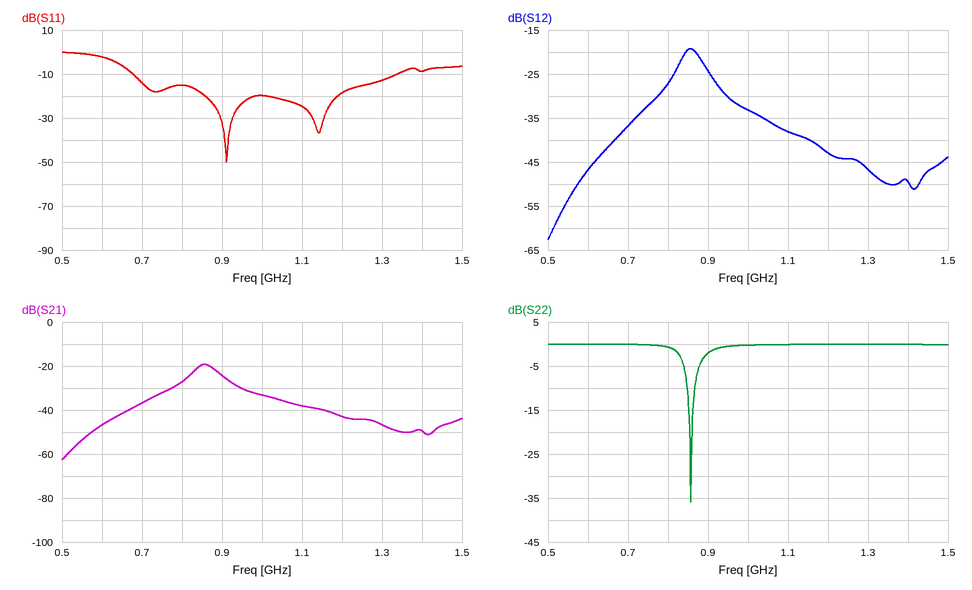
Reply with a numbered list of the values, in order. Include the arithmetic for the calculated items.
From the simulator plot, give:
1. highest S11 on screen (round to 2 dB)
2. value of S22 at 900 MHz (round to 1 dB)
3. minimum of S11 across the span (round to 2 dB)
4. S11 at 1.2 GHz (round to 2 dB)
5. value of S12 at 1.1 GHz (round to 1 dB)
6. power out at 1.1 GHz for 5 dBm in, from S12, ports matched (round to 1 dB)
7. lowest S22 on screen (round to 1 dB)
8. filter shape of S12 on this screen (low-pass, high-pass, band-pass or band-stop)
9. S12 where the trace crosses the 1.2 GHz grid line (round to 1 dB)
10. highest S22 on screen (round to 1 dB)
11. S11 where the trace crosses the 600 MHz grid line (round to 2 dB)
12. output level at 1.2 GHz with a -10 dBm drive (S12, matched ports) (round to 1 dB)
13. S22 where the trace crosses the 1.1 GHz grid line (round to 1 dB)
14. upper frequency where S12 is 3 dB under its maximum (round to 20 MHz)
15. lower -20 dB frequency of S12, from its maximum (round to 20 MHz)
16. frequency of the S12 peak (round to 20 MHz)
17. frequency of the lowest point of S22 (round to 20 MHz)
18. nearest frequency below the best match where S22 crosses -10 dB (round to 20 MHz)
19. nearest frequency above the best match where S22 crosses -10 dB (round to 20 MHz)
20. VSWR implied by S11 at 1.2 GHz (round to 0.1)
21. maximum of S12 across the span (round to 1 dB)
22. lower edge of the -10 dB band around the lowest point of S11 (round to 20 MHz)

1. 0 dB
2. -2 dB
3. -50 dB
4. -18 dB
5. -38 dB
6. 5 dBm + (-38 dB) = -33 dBm
7. -36 dB
8. band-pass
9. -43 dB
10. 0 dB
11. -2 dB
12. -10 dBm + (-43 dB) = -53 dBm
13. 0 dB
14. 880 MHz
15. 680 MHz
16. 860 MHz
17. 860 MHz
18. 840 MHz
19. 860 MHz
20. |Γ| = 10^(-18/20) = 0.1259; VSWR = (1 + 0.1259)/(1 − 0.1259) ≈ 1.3
21. -19 dB
22. 680 MHz
